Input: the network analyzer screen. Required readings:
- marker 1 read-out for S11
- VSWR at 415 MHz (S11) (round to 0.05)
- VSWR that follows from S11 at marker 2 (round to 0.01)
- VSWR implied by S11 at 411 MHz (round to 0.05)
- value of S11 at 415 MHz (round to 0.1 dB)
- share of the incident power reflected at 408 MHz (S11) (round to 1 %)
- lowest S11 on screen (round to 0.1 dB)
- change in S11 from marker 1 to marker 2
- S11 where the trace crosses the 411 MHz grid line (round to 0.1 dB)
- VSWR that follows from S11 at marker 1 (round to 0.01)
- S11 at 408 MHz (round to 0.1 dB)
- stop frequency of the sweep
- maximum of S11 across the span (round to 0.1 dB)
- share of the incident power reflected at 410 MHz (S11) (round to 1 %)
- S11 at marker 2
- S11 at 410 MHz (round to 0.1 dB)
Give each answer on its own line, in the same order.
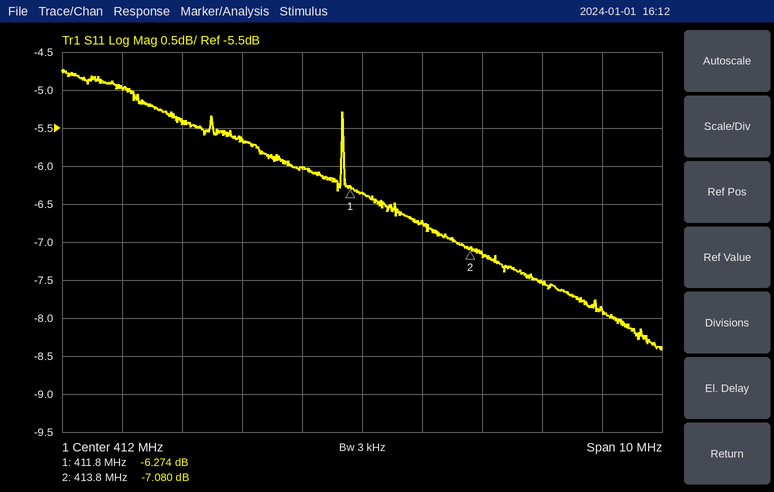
-6.274 dB
2.45
2.59
3.00
-7.5 dB
32 %
-8.4 dB
-0.806 dB
-6.0 dB
2.89
-5.0 dB
417 MHz
-4.7 dB
27 %
-7.080 dB
-5.7 dB
